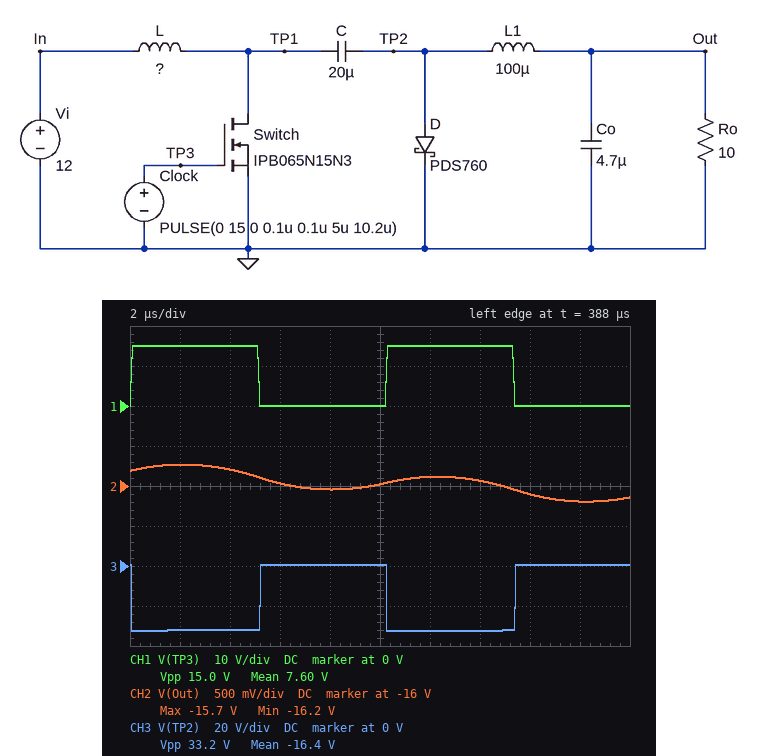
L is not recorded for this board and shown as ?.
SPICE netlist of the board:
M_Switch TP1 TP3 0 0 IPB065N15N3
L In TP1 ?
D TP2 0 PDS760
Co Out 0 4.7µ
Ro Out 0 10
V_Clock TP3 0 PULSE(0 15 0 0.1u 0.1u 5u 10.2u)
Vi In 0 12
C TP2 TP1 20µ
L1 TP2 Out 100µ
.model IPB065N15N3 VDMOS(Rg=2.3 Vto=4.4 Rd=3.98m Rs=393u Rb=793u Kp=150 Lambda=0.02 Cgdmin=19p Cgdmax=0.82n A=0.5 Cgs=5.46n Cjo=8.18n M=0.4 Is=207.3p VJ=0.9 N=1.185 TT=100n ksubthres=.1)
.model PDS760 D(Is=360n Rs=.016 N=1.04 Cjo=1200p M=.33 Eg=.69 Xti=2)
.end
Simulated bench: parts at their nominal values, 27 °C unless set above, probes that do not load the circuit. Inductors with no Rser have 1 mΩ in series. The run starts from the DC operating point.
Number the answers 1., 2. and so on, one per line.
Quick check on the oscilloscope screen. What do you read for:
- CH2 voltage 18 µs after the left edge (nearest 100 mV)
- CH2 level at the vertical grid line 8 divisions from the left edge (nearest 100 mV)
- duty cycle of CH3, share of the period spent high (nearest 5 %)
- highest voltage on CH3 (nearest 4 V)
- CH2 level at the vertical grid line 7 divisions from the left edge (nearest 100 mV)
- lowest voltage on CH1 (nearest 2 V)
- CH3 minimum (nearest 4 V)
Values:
1. -16.2 V
2. -16.1 V
3. 50 %
4. 0 V
5. -15.9 V
6. 0 V
7. -32 V
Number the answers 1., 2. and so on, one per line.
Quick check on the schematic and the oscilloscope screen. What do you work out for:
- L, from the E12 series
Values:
1. 220 µH
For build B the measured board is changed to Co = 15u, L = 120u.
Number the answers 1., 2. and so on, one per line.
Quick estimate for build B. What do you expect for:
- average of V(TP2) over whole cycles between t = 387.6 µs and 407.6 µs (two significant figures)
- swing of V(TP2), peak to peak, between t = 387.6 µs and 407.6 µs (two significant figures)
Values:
1. -17 V
2. 34 V
